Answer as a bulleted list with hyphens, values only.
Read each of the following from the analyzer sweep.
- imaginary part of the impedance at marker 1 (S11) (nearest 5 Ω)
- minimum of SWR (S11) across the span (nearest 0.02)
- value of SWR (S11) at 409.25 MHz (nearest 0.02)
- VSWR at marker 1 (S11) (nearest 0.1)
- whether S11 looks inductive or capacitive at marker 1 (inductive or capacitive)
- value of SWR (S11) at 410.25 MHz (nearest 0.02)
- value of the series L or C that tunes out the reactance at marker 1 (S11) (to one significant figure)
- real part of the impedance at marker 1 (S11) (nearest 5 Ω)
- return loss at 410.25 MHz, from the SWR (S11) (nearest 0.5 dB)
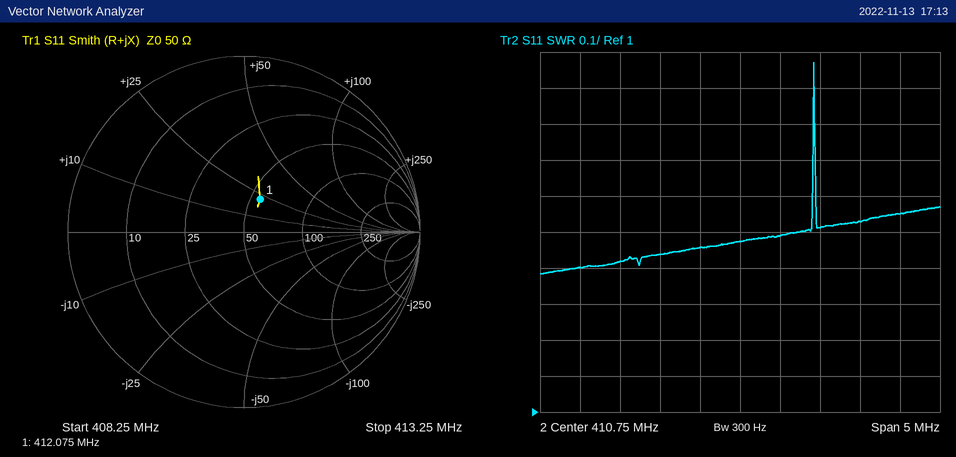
- +20 Ω
- 1.38
- 1.42
- 1.5
- inductive
- 1.46
- 20 pF
- 55 Ω
- 14.5 dB
